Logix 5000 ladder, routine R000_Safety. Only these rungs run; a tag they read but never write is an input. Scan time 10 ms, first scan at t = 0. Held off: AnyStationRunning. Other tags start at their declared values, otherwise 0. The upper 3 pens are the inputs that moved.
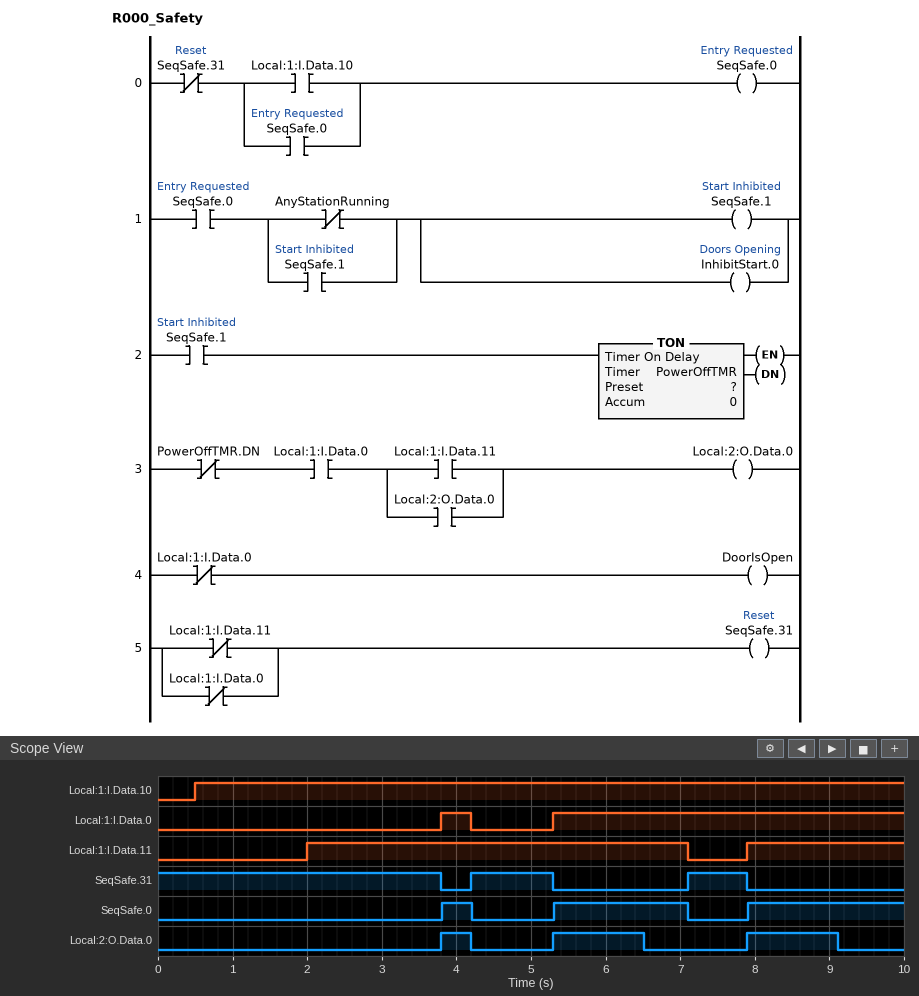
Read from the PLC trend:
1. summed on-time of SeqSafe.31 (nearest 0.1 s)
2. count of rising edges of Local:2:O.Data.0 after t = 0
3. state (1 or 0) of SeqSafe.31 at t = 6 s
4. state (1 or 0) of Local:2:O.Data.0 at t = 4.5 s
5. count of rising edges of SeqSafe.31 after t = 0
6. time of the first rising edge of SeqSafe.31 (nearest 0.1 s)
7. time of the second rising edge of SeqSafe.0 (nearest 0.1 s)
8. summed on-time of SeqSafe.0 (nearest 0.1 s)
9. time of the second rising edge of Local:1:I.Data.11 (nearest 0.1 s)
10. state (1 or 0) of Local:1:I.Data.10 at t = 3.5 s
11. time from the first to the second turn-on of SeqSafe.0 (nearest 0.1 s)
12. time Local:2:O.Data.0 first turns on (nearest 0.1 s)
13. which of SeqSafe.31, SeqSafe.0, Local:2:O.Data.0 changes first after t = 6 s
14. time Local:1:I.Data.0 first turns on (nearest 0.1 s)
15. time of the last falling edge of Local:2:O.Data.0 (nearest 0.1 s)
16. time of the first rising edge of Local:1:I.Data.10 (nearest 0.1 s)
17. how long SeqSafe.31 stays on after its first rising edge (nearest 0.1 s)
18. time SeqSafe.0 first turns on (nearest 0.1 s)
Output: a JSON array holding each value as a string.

["5.7 s", "3", "0", "0", "2", "4.2 s", "5.3 s", "4.3 s", "7.9 s", "1", "1.5 s", "3.8 s", "Local:2:O.Data.0", "3.8 s", "9.1 s", "0.5 s", "1.1 s", "3.8 s"]
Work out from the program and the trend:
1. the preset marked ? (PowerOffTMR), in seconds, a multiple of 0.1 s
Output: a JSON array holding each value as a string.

["1.2 s"]
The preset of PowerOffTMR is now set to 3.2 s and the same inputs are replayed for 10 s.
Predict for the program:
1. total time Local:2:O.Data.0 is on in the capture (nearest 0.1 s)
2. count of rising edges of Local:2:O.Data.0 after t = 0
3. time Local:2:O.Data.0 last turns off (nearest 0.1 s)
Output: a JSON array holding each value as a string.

["5.1 s", "2", "4.2 s"]
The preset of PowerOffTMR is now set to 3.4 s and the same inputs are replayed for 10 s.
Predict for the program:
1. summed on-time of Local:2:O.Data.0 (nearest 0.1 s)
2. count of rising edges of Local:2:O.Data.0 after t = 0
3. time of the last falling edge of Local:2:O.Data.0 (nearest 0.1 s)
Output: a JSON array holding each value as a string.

["5.1 s", "2", "4.2 s"]
